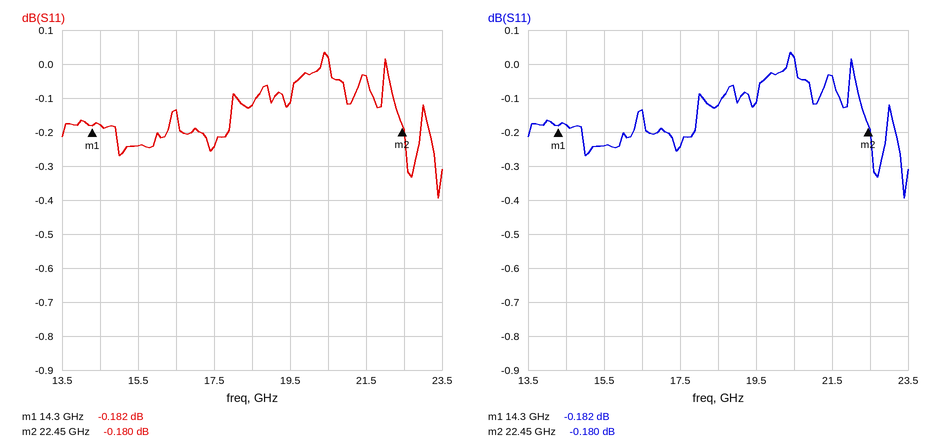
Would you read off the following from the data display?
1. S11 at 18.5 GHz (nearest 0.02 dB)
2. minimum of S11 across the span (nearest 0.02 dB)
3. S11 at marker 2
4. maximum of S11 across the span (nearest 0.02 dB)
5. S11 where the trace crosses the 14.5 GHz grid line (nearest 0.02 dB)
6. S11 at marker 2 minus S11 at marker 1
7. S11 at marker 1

-0.12 dB
-0.40 dB
-0.180 dB
0.04 dB
-0.18 dB
0.002 dB
-0.182 dB
